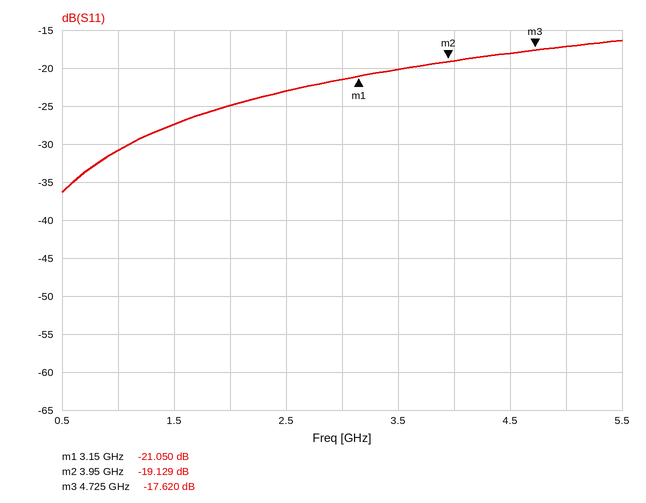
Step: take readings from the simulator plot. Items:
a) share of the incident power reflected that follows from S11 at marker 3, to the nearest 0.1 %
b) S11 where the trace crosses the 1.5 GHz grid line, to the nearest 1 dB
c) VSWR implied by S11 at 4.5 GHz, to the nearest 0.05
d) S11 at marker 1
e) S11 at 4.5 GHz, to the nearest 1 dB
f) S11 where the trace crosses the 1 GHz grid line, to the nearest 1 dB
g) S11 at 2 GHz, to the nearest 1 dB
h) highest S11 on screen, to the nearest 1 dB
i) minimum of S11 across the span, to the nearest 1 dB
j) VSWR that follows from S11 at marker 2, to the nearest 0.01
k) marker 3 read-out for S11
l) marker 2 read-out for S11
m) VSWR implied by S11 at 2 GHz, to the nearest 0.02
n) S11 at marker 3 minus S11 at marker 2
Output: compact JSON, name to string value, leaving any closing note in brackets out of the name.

{"share of the incident power reflected that follows from S11 at marker 3, to the nearest 0.1 %": "1.7 %", "S11 where the trace crosses the 1.5 GHz grid line, to the nearest 1 dB": "-27 dB", "VSWR implied by S11 at 4.5 GHz, to the nearest 0.05": "1.30", "S11 at marker 1": "-21.050 dB", "S11 at 4.5 GHz, to the nearest 1 dB": "-18 dB", "S11 where the trace crosses the 1 GHz grid line, to the nearest 1 dB": "-31 dB", "S11 at 2 GHz, to the nearest 1 dB": "-25 dB", "highest S11 on screen, to the nearest 1 dB": "-16 dB", "minimum of S11 across the span, to the nearest 1 dB": "-36 dB", "VSWR that follows from S11 at marker 2, to the nearest 0.01": "1.25", "marker 3 read-out for S11": "-17.620 dB", "marker 2 read-out for S11": "-19.129 dB", "VSWR implied by S11 at 2 GHz, to the nearest 0.02": "1.12", "S11 at marker 3 minus S11 at marker 2": "1.509 dB"}
